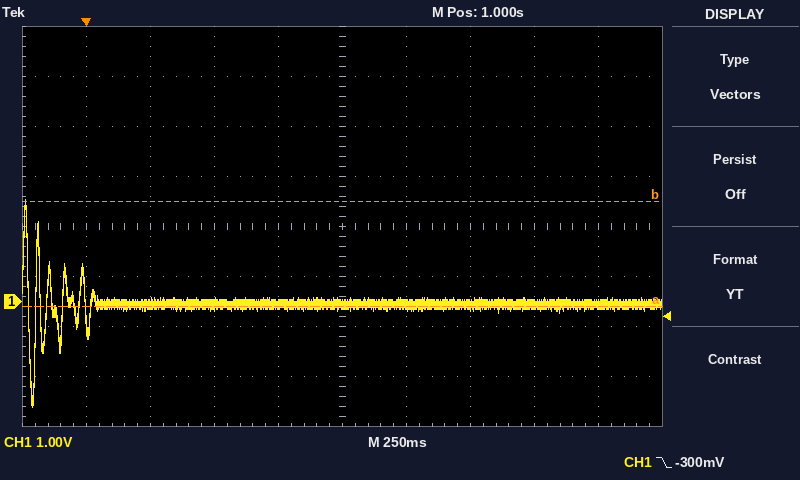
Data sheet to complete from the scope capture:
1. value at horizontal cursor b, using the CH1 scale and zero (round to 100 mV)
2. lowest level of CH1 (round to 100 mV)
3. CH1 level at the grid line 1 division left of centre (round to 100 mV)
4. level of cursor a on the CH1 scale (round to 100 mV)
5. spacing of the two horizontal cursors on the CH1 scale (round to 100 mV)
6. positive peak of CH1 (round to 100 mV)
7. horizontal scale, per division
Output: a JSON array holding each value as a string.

["2.0 V", "-2.1 V", "-100 mV", "-100 mV", "2.1 V", "2.0 V", "250 ms"]
